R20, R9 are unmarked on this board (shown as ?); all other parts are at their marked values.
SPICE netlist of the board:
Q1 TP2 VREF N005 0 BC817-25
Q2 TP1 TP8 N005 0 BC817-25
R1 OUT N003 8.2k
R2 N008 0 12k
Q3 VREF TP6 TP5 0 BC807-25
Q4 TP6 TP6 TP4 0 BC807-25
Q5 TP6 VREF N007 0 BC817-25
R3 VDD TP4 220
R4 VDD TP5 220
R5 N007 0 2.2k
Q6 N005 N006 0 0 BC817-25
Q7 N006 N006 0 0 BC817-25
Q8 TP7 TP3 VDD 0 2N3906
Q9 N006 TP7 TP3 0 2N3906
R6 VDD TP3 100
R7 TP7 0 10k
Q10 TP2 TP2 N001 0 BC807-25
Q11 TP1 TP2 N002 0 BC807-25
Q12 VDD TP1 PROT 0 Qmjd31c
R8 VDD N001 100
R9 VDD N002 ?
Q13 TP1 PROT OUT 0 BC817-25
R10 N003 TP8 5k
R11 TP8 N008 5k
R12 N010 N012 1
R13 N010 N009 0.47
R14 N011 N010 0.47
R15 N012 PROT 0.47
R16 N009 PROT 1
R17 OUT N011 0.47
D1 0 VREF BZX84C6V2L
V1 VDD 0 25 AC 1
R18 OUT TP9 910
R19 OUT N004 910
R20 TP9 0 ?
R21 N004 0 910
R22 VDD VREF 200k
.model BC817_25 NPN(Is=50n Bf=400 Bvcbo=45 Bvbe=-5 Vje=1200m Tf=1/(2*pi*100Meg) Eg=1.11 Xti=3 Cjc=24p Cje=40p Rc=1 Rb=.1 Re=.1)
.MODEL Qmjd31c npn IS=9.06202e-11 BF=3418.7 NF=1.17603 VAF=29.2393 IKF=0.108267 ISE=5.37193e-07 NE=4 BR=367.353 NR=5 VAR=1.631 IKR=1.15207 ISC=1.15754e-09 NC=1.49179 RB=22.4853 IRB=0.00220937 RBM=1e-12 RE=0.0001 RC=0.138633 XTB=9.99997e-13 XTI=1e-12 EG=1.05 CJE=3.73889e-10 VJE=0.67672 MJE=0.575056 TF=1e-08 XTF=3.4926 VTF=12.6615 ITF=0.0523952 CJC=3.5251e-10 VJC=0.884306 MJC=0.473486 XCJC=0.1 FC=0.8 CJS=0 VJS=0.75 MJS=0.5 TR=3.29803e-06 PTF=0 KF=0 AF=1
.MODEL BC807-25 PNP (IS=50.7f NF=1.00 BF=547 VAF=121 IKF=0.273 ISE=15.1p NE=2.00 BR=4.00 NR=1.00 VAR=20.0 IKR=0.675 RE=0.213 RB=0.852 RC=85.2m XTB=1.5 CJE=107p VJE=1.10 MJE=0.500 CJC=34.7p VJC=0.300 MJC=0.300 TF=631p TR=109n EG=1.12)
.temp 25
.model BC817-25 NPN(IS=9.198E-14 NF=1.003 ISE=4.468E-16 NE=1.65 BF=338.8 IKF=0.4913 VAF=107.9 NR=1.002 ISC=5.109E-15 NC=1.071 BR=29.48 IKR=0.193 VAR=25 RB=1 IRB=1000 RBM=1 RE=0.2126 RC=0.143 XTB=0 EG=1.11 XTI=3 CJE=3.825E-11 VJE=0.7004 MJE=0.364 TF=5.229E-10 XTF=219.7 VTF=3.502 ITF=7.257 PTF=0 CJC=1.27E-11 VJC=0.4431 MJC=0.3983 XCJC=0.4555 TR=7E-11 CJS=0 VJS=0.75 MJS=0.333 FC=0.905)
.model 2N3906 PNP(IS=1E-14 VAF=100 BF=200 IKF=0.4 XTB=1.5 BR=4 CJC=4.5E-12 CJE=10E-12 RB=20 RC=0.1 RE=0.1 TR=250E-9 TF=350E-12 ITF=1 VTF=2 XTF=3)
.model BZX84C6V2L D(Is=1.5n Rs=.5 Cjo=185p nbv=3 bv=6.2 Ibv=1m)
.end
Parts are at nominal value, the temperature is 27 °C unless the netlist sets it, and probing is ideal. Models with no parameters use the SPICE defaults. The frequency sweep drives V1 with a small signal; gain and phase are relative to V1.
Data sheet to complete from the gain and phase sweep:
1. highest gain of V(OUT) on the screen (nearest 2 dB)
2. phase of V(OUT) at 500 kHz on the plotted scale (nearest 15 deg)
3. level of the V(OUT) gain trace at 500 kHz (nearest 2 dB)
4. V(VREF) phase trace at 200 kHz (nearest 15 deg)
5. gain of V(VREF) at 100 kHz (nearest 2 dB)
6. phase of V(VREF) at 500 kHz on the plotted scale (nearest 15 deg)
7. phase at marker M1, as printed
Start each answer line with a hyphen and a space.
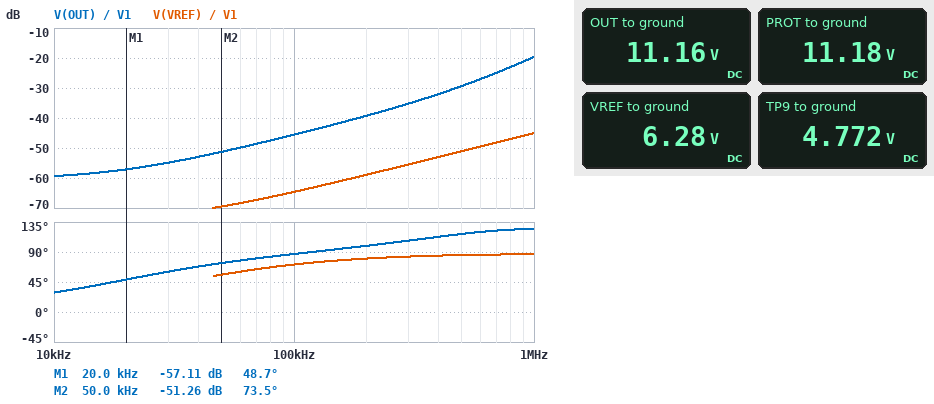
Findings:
- -20 dB
- 120 deg
- -30 dB
- 75 deg
- -64 dB
- 90 deg
- 48.7 deg
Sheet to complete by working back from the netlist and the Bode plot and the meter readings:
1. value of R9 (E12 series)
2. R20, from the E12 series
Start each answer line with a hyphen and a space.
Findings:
- 330 Ω
- 680 Ω
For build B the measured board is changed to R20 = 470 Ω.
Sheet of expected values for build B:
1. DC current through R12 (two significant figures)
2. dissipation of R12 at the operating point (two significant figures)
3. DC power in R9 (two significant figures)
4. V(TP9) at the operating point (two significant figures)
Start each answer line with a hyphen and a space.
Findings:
- 7.3 mA
- 53 µW
- 1.0 mW
- 3.8 V
